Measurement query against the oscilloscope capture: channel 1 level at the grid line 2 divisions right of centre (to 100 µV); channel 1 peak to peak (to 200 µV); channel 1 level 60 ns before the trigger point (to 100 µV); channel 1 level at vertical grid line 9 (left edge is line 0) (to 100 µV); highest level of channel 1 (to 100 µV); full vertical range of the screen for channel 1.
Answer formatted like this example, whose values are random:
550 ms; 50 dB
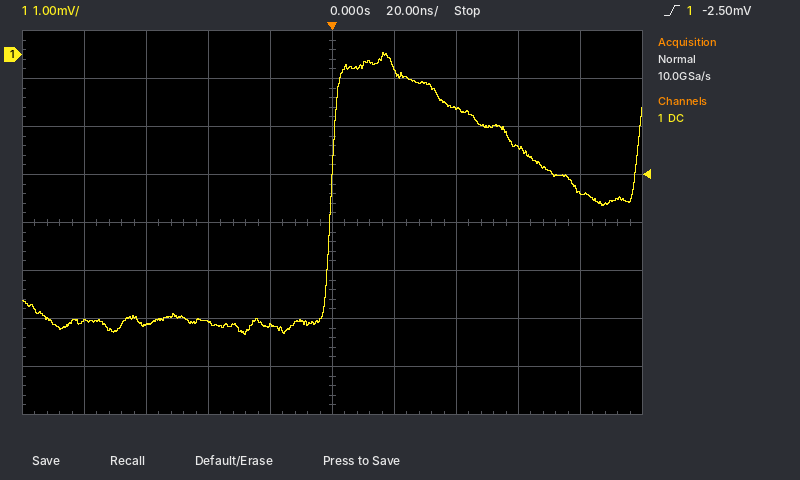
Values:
-1.1 mV; 5.8 mV; -5.6 mV; -2.9 mV; 0.0 mV; 8 mV
